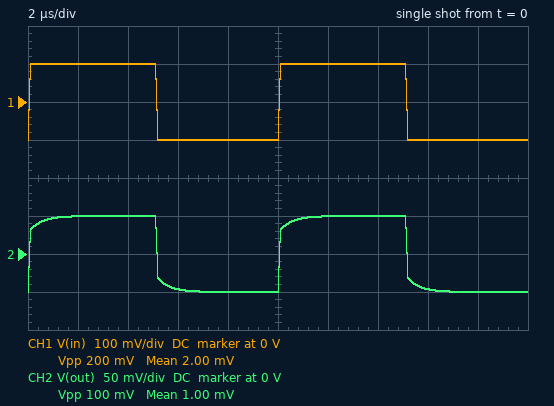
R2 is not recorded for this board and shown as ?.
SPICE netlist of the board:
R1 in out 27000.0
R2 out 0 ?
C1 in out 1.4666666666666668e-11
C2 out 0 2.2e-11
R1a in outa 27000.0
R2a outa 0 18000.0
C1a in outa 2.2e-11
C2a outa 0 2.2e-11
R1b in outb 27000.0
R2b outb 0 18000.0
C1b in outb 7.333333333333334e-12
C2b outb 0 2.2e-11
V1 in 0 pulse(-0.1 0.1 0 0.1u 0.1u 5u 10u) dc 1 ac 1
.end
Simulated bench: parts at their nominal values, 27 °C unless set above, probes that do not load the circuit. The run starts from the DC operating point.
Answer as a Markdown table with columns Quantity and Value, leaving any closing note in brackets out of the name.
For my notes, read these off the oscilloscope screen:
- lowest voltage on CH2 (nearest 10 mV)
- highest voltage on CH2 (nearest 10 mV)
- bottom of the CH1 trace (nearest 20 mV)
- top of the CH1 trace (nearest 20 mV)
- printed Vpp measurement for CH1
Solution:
| Quantity | Value |
|---|---|
| lowest voltage on CH2 | -50 mV |
| highest voltage on CH2 | 50 mV |
| bottom of the CH1 trace | -100 mV |
| top of the CH1 trace | 100 mV |
| printed Vpp measurement for CH1 | 200 mV |
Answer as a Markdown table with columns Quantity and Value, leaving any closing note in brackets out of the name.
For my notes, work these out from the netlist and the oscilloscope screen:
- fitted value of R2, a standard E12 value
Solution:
| Quantity | Value |
|---|---|
| fitted value of R2, a standard E12 value | 27 kΩ |
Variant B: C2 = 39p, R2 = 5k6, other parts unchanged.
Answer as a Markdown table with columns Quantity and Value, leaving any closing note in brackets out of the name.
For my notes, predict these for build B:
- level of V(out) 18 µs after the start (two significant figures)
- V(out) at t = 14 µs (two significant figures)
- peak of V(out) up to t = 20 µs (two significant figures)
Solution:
| Quantity | Value |
|---|---|
| level of V(out) 18 µs after the start | -17 mV |
| V(out) at t = 14 µs | 17 mV |
| peak of V(out) up to t = 20 µs | 34 mV |
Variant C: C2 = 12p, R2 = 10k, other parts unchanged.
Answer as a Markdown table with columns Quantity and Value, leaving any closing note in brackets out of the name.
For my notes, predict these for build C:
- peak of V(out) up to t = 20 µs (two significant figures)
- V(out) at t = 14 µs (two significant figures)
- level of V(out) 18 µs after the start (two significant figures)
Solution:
| Quantity | Value |
|---|---|
| peak of V(out) up to t = 20 µs | 71 mV |
| V(out) at t = 14 µs | 27 mV |
| level of V(out) 18 µs after the start | -27 mV |
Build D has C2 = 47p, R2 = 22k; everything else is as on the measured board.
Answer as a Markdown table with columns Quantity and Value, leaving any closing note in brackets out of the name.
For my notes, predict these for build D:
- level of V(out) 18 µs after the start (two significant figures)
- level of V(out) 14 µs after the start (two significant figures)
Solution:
| Quantity | Value |
|---|---|
| level of V(out) 18 µs after the start | -44 mV |
| level of V(out) 14 µs after the start | 45 mV |
